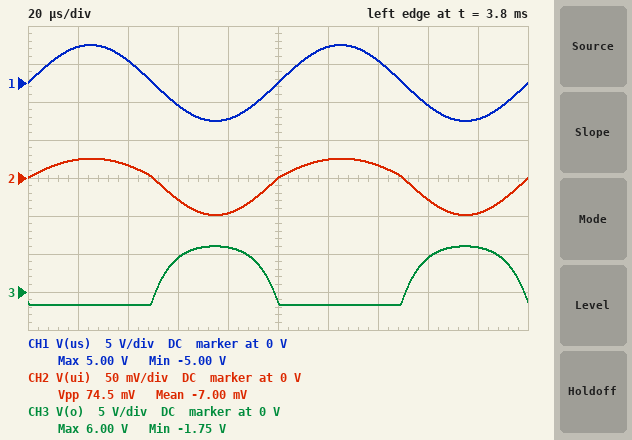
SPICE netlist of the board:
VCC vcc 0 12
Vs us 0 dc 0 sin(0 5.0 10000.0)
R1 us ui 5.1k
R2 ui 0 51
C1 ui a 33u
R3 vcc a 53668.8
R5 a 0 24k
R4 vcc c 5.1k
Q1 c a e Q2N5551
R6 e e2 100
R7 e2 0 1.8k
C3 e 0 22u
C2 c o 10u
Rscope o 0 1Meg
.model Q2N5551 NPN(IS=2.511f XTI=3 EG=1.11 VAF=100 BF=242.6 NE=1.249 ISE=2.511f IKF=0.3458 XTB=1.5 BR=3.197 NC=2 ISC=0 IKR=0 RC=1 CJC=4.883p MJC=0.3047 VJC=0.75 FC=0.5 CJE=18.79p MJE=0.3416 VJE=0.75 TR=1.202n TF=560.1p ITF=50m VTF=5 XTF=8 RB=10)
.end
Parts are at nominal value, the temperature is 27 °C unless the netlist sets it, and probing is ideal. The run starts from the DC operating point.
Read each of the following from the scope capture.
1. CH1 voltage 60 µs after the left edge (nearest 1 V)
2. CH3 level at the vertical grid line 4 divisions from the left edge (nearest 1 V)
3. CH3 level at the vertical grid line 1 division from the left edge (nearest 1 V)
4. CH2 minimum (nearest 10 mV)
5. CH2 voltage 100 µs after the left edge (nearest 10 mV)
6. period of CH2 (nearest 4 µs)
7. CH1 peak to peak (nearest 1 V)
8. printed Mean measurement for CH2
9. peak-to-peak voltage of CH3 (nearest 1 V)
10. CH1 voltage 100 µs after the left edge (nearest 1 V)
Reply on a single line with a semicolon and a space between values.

-3 V; 6 V; -2 V; -50 mV; 0 V; 100 µs; 10 V; -7.00 mV; 8 V; 0 V
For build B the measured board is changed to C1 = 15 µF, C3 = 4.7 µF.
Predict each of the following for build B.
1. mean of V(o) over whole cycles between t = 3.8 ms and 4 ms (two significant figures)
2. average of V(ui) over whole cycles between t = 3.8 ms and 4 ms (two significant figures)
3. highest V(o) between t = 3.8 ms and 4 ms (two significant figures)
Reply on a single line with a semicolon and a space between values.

1.1 V; -7.4 mV; 5.9 V
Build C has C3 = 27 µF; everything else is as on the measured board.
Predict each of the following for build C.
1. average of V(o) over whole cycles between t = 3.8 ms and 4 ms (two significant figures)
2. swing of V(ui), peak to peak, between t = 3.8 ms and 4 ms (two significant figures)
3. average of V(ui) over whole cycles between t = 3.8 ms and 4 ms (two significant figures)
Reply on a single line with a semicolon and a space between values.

1.3 V; 75 mV; -6.8 mV
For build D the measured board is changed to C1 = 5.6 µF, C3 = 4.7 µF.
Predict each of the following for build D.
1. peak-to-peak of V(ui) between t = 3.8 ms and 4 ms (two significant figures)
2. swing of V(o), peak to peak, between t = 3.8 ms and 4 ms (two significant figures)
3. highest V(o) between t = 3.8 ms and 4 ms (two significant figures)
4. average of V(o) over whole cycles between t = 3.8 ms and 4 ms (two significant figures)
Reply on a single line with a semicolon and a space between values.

76 mV; 8.0 V; 6.1 V; 1.4 V
